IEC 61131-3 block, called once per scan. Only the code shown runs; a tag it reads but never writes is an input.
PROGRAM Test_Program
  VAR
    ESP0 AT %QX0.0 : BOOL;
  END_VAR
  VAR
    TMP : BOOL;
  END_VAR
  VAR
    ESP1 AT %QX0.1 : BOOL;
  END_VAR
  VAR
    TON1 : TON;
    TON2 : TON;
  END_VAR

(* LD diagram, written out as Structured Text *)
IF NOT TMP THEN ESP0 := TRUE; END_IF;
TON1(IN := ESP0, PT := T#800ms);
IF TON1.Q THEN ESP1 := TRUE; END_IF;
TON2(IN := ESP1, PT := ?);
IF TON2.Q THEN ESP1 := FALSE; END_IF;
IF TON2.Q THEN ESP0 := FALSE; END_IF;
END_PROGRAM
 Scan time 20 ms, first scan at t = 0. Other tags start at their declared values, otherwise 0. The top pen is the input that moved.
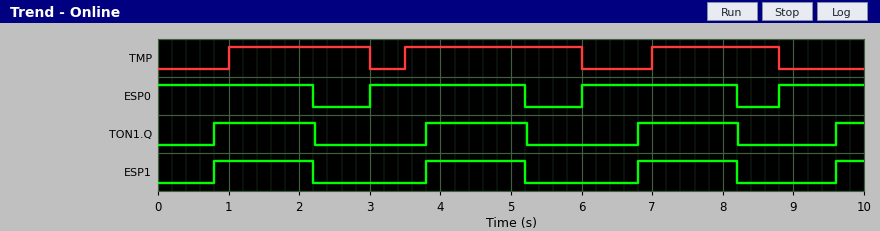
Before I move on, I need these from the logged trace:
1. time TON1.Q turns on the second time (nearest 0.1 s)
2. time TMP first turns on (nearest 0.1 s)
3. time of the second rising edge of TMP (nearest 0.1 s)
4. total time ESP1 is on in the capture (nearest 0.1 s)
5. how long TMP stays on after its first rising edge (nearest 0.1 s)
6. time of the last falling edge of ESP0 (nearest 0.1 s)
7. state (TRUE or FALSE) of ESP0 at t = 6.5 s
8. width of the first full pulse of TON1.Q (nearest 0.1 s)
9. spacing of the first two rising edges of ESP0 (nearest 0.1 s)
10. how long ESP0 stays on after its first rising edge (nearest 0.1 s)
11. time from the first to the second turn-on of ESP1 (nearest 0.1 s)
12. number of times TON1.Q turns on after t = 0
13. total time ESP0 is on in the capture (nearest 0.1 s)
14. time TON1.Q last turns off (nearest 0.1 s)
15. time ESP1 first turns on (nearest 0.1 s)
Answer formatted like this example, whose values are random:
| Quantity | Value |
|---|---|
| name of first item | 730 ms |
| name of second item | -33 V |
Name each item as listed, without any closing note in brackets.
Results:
| Quantity | Value |
|---|---|
| time TON1.Q turns on the second time | 3.8 s |
| time TMP first turns on | 1.0 s |
| time of the second rising edge of TMP | 3.5 s |
| total time ESP1 is on in the capture | 4.6 s |
| how long TMP stays on after its first rising edge | 2.0 s |
| time of the last falling edge of ESP0 | 8.2 s |
| state (TRUE or FALSE) of ESP0 at t = 6.5 s | TRUE |
| width of the first full pulse of TON1.Q | 1.4 s |
| spacing of the first two rising edges of ESP0 | 3.0 s |
| how long ESP0 stays on after its first rising edge | 2.2 s |
| time from the first to the second turn-on of ESP1 | 3.0 s |
| number of times TON1.Q turns on after t = 0 | 4 |
| total time ESP0 is on in the capture | 7.8 s |
| time TON1.Q last turns off | 8.2 s |
| time ESP1 first turns on | 0.8 s |
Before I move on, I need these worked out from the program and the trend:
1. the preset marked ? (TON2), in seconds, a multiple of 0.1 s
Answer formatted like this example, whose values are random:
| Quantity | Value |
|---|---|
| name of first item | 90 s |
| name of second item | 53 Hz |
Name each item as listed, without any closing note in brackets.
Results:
| Quantity | Value |
|---|---|
| the preset marked ? (TON2), in seconds, a multiple of 0.1 s | 1.4 s |
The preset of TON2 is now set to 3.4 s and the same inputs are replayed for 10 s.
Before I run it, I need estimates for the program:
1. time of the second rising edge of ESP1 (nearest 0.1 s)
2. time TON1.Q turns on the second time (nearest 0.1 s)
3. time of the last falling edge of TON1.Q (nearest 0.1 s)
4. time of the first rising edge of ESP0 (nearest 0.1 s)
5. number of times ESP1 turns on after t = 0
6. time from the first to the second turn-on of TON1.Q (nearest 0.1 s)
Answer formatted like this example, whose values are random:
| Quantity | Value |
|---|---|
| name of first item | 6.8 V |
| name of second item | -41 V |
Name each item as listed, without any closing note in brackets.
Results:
| Quantity | Value |
|---|---|
| time of the second rising edge of ESP1 | 6.8 s |
| time TON1.Q turns on the second time | 6.8 s |
| time of the last falling edge of TON1.Q | 4.2 s |
| time of the first rising edge of ESP0 | 6.0 s |
| number of times ESP1 turns on after t = 0 | 2 |
| time from the first to the second turn-on of TON1.Q | 6.0 s |
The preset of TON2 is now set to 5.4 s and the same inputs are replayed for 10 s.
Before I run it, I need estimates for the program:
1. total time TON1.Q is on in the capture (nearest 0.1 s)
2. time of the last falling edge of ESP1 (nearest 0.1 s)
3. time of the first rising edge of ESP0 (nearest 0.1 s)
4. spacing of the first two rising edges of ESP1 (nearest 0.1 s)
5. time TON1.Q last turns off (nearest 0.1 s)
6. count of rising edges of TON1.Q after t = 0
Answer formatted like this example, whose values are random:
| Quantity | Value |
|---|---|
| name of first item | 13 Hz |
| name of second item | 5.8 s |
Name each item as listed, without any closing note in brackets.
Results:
| Quantity | Value |
|---|---|
| total time TON1.Q is on in the capture | 6.6 s |
| time of the last falling edge of ESP1 | 6.2 s |
| time of the first rising edge of ESP0 | 8.8 s |
| spacing of the first two rising edges of ESP1 | 8.8 s |
| time TON1.Q last turns off | 7.0 s |
| count of rising edges of TON1.Q after t = 0 | 2 |
